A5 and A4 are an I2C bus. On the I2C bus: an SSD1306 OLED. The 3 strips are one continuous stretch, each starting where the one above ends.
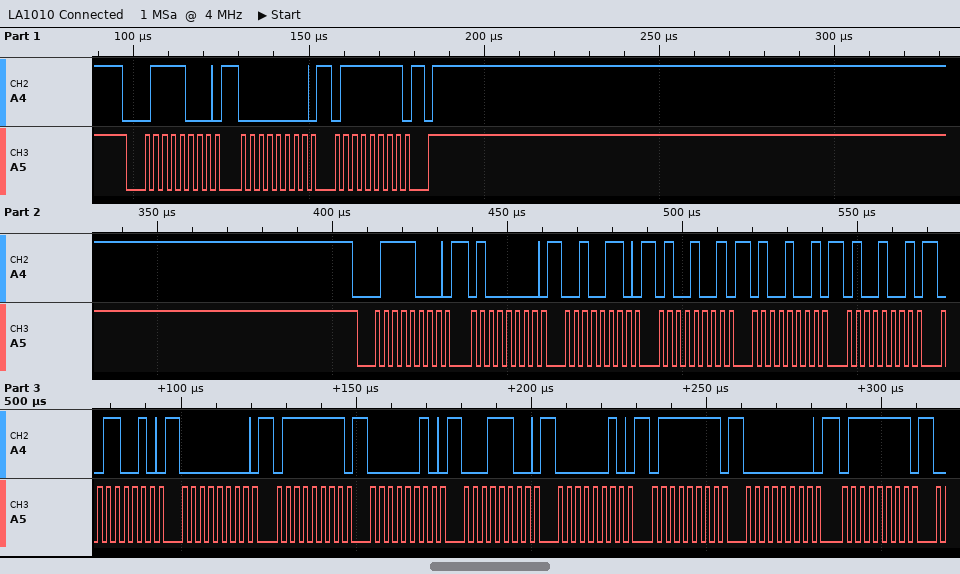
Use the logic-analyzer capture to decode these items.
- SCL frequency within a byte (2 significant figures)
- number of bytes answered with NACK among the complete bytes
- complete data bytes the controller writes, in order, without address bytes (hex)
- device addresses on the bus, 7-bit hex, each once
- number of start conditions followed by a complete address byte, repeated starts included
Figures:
400 kHz
0
00 7F 40 26 49 49 49 32 00 7F 02 1C 02 7F 00 7F
0x3C
2
